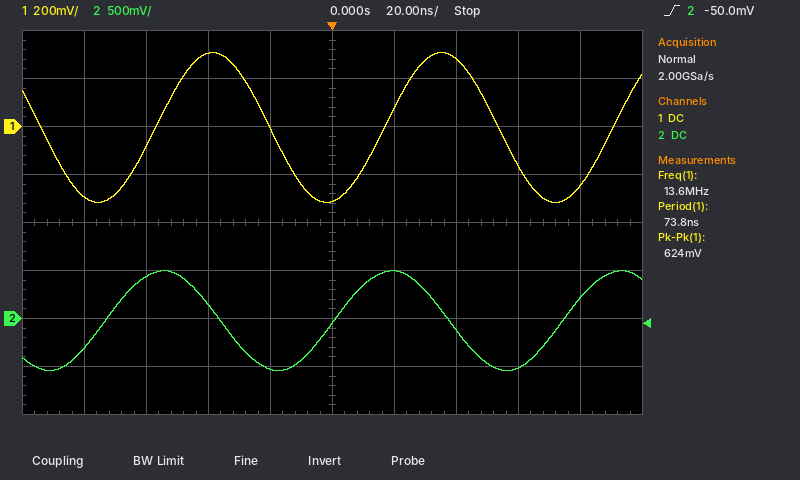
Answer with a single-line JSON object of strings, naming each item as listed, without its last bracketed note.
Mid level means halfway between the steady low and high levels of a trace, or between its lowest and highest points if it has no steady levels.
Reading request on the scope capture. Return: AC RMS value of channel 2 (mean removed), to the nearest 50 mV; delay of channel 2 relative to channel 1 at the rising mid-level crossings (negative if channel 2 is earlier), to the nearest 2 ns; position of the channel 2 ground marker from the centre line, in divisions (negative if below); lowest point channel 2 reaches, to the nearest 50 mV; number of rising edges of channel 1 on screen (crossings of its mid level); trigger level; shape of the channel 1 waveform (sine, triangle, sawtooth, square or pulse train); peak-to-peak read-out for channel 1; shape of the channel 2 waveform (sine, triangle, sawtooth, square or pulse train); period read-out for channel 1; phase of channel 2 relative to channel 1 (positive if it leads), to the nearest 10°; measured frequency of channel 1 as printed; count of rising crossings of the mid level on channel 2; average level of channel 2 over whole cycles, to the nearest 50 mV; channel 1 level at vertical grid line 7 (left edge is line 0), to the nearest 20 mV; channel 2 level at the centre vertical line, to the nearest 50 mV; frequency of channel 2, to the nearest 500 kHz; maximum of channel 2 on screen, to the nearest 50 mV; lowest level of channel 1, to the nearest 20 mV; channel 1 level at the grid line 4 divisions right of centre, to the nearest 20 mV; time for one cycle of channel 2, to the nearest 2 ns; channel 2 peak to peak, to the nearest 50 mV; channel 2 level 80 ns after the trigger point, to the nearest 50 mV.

{"AC RMS value of channel 2 (mean removed), to the nearest 50 mV": "350 mV", "delay of channel 2 relative to channel 1 at the rising mid-level crossings (negative if channel 2 is earlier), to the nearest 2 ns": "-16 ns", "position of the channel 2 ground marker from the centre line, in divisions": "-2.0 div", "lowest point channel 2 reaches, to the nearest 50 mV": "-550 mV", "number of rising edges of channel 1 on screen": "3", "trigger level": "-50.0 mV", "shape of the channel 1 waveform": "sine", "peak-to-peak read-out for channel 1": "624 mV", "shape of the channel 2 waveform": "sine", "period read-out for channel 1": "73.8 ns", "phase of channel 2 relative to channel 1 (positive if it leads), to the nearest 10°": "+80°", "measured frequency of channel 1 as printed": "13.6 MHz", "count of rising crossings of the mid level on channel 2": "3", "average level of channel 2 over whole cycles, to the nearest 50 mV": "0 mV", "channel 1 level at vertical grid line 7 (left edge is line 0), to the nearest 20 mV": "280 mV", "channel 2 level at the centre vertical line, to the nearest 50 mV": "-50 mV", "frequency of channel 2, to the nearest 500 kHz": "13.5 MHz", "maximum of channel 2 on screen, to the nearest 50 mV": "500 mV", "lowest level of channel 1, to the nearest 20 mV": "-320 mV", "channel 1 level at the grid line 4 divisions right of centre, to the nearest 20 mV": "-240 mV", "time for one cycle of channel 2, to the nearest 2 ns": "74 ns", "channel 2 peak to peak, to the nearest 50 mV": "1.05 V", "channel 2 level 80 ns after the trigger point, to the nearest 50 mV": "200 mV"}
